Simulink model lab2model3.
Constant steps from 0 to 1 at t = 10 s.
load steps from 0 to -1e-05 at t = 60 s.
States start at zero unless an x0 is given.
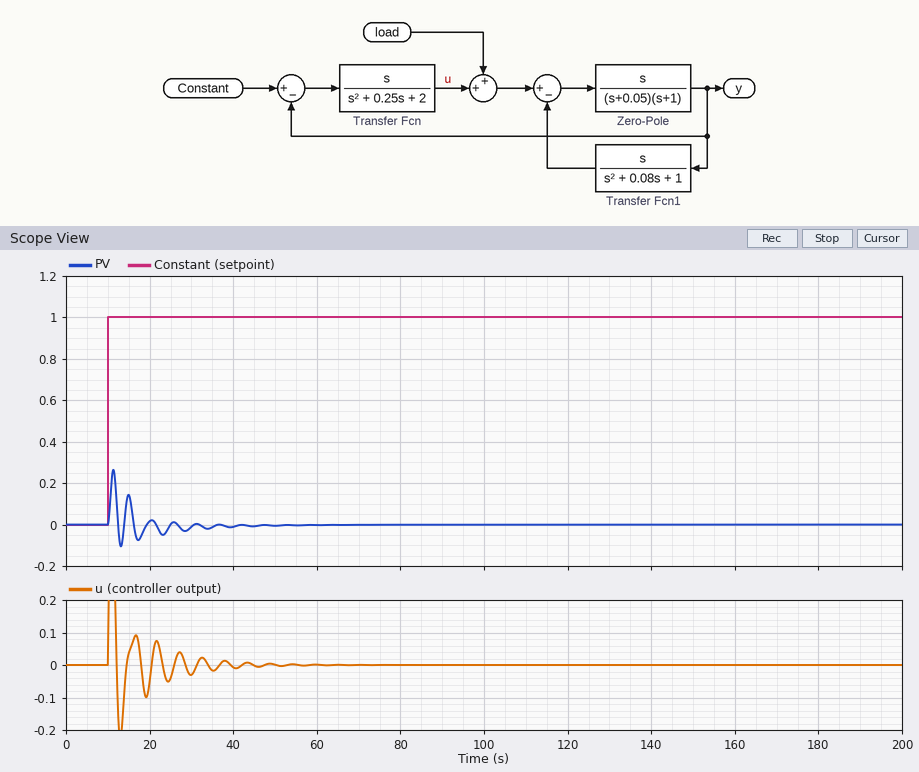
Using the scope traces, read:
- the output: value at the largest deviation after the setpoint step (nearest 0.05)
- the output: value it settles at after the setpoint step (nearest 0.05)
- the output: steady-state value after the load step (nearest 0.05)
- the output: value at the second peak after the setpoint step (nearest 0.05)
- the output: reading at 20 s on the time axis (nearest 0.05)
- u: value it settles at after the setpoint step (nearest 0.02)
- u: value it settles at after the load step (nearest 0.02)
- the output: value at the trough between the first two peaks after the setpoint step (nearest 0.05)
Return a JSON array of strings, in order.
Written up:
["0.25", "0.00", "0.00", "0.15", "0.00", "0.00", "0.00", "-0.10"]
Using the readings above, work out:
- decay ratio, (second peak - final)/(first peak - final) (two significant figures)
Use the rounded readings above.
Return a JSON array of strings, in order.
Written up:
["0.60"]
